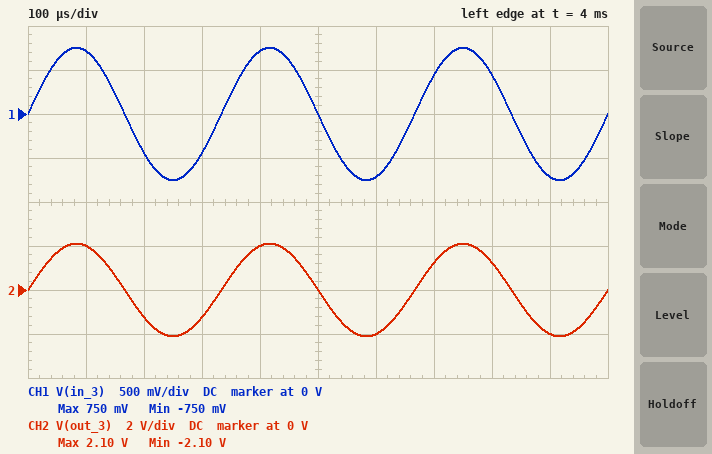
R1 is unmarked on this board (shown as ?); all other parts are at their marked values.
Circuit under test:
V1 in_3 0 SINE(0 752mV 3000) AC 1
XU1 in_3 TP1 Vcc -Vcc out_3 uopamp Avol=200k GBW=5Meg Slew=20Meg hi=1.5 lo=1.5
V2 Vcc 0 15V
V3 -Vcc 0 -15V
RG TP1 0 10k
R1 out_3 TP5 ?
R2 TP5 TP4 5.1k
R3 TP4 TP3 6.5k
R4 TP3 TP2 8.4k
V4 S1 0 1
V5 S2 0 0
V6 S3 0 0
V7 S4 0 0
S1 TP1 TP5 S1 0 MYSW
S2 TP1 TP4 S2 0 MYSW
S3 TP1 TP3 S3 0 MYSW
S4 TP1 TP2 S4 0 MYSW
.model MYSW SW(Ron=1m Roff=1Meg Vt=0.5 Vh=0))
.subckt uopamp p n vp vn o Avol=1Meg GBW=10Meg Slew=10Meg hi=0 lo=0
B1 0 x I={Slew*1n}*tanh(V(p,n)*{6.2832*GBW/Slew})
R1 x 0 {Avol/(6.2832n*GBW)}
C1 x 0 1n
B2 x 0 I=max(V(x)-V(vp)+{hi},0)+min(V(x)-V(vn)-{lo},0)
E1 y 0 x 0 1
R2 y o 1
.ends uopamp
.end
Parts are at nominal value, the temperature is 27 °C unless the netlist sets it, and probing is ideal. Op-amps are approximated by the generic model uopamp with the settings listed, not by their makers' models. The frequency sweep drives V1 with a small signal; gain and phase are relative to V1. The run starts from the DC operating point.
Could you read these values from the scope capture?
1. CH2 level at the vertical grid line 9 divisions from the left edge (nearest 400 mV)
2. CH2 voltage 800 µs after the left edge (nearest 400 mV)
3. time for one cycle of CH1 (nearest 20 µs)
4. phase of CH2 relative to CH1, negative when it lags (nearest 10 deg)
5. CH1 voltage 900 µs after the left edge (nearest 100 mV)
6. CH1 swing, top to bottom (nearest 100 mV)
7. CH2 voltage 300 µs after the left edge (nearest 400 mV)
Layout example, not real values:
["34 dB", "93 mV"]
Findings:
["-2.0 V", "1.2 V", "340 µs", "0 deg", "-700 mV", "1.5 V", "-1.2 V"]
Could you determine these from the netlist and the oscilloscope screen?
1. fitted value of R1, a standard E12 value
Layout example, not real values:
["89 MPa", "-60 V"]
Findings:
["18 kΩ"]
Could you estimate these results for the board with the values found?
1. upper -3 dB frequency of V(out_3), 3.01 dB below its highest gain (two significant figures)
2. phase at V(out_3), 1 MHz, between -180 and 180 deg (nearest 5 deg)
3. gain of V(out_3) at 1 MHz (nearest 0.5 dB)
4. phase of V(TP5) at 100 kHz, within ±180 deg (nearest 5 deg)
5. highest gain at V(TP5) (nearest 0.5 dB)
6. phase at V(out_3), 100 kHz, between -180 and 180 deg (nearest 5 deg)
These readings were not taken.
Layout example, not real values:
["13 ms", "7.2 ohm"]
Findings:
["180 kHz", "-80 deg", "14.0 dB", "-30 deg", "28.5 dB", "-30 deg"]
